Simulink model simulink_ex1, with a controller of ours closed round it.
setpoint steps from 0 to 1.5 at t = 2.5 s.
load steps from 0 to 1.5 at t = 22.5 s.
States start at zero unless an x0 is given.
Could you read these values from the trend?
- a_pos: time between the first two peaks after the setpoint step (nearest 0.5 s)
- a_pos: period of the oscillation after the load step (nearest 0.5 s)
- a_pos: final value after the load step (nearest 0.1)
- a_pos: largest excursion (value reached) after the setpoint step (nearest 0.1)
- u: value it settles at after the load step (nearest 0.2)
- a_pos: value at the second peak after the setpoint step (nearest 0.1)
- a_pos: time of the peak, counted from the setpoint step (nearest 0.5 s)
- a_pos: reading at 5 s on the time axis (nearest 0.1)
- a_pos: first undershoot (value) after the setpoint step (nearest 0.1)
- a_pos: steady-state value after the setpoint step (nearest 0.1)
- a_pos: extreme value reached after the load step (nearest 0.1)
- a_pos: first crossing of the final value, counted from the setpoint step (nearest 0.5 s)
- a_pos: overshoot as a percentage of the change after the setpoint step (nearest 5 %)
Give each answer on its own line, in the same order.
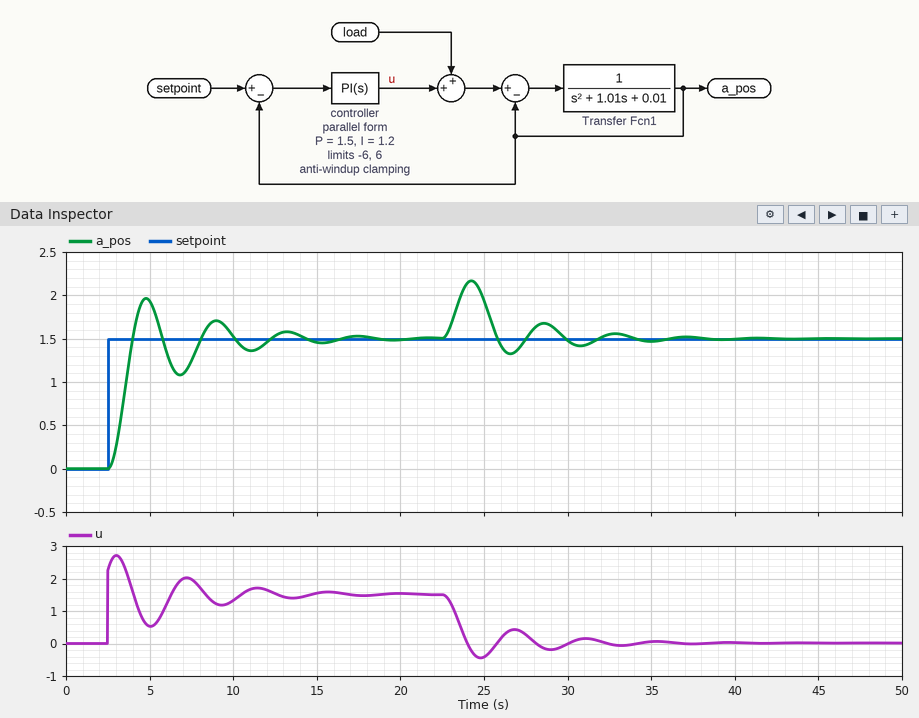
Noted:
4.0 s
4.5 s
1.5
2.0
0.0
1.7
2.5 s
1.9
1.1
1.5
2.2
1.5 s
30 %
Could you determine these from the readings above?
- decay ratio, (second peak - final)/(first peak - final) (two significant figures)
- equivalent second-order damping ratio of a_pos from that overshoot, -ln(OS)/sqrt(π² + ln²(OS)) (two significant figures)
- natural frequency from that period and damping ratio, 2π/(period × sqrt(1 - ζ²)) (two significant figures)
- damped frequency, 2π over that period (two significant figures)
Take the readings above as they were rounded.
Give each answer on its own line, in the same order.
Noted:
0.40
0.36
1.7 rad/s
1.6 rad/s
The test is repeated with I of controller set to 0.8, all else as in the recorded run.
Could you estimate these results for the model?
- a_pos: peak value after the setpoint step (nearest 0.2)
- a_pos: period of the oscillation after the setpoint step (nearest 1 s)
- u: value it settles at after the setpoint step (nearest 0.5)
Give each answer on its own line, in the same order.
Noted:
1.8
4 s
1.5
